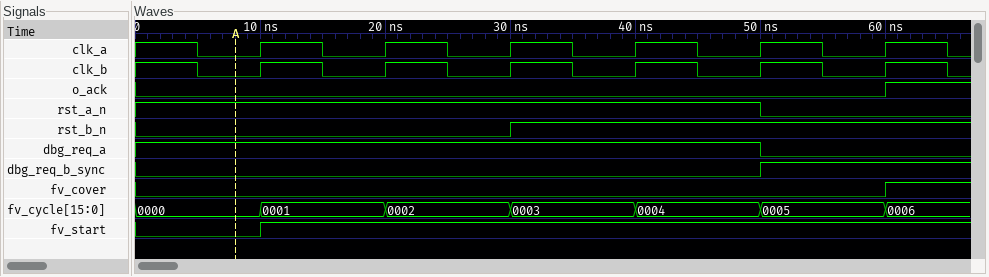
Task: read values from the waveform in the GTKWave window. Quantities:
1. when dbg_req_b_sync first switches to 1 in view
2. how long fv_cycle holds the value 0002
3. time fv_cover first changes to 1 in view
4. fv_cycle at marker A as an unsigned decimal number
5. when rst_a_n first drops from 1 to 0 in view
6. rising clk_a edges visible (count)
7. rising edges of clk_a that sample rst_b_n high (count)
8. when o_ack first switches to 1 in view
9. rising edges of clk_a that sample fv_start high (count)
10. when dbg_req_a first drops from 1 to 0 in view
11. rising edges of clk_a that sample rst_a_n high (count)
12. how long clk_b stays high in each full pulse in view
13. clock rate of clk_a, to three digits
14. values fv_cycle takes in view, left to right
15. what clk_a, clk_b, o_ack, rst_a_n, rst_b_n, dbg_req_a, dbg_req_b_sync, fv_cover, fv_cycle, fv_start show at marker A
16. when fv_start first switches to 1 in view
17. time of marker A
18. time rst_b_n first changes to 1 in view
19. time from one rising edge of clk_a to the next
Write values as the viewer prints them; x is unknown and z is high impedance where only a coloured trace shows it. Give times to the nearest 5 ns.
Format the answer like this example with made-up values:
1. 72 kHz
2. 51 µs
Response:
1. 50 ns
2. 10 ns
3. 60 ns
4. 0
5. 50 ns
6. 6
7. 3
8. 60 ns
9. 5
10. 50 ns
11. 5
12. 5 ns, 5 ns, 5 ns, 5 ns, 5 ns, 5 ns
13. 100 MHz
14. 0000, 0001, 0002, 0003, 0004, 0005, 0006
15. clk_a=0, clk_b=0, o_ack=0, rst_a_n=1, rst_b_n=0, dbg_req_a=1, dbg_req_b_sync=0, fv_cover=0, fv_cycle=0000, fv_start=0
16. 10 ns
17. 10 ns
18. 30 ns
19. 10 ns
